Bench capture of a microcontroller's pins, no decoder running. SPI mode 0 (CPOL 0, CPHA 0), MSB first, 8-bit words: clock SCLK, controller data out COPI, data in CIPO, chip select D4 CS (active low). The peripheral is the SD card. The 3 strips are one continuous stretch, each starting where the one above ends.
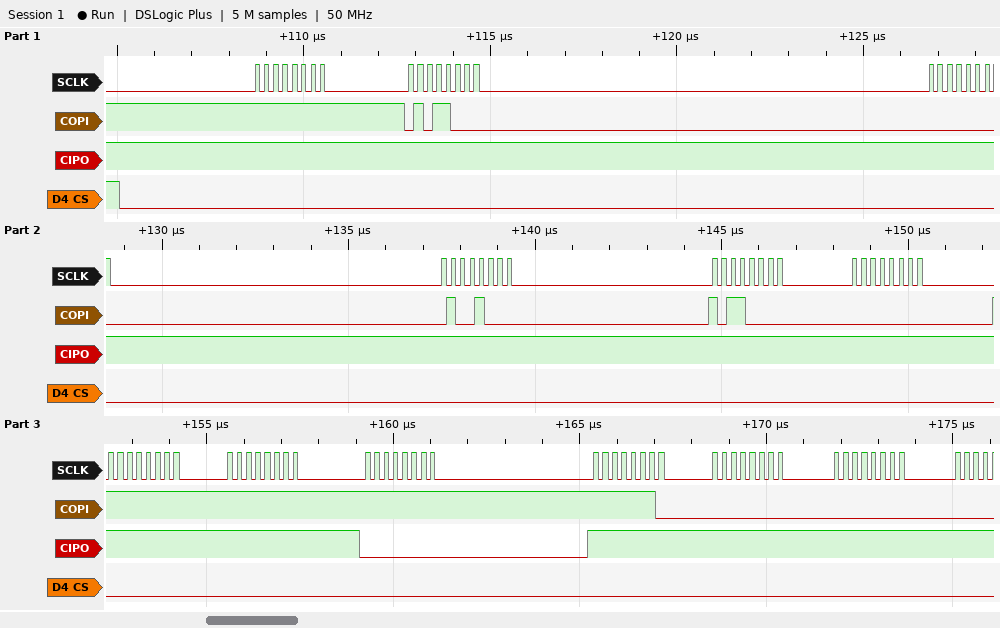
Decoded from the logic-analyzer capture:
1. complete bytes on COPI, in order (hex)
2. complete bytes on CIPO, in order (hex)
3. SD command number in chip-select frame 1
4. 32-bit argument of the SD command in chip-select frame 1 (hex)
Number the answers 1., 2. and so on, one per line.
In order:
1. 0xFF 0x58 0x00 0x48 0xB0 0x00 0xFF 0xFF 0xFF 0xFE 0x00 0x00
2. 0xFF 0xFF 0xFF 0xFF 0xFF 0xFF 0xFF 0xFF 0x00 0xFF 0xFF 0xFF
3. CMD24
4. 0x0048B000
